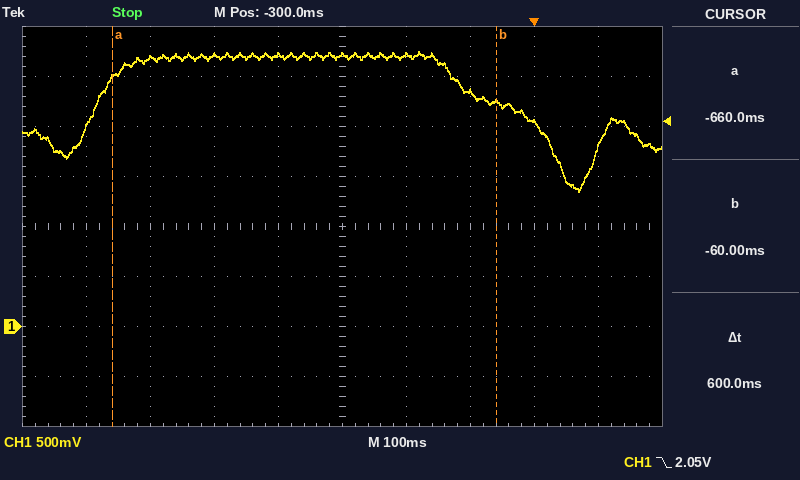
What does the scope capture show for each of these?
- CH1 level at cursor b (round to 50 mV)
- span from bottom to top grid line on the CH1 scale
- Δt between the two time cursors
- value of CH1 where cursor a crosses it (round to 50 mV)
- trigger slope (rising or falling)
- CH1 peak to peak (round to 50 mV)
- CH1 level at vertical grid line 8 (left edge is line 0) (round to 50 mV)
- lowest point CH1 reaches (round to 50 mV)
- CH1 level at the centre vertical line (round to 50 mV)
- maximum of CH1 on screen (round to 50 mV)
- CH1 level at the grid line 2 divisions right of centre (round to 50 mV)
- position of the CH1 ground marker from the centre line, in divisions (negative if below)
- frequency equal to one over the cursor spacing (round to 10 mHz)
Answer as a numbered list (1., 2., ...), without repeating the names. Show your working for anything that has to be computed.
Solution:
1. 2.25 V
2. 4 V
3. 600 ms
4. 2.50 V
5. falling
6. 2.75 V − (1.35 V) = 1.40 V
7. 2.05 V
8. 1.35 V
9. 2.70 V
10. 2.75 V
11. 2.35 V
12. -2.0 div
13. 1 / 600 ms ≈ 1.67 Hz
